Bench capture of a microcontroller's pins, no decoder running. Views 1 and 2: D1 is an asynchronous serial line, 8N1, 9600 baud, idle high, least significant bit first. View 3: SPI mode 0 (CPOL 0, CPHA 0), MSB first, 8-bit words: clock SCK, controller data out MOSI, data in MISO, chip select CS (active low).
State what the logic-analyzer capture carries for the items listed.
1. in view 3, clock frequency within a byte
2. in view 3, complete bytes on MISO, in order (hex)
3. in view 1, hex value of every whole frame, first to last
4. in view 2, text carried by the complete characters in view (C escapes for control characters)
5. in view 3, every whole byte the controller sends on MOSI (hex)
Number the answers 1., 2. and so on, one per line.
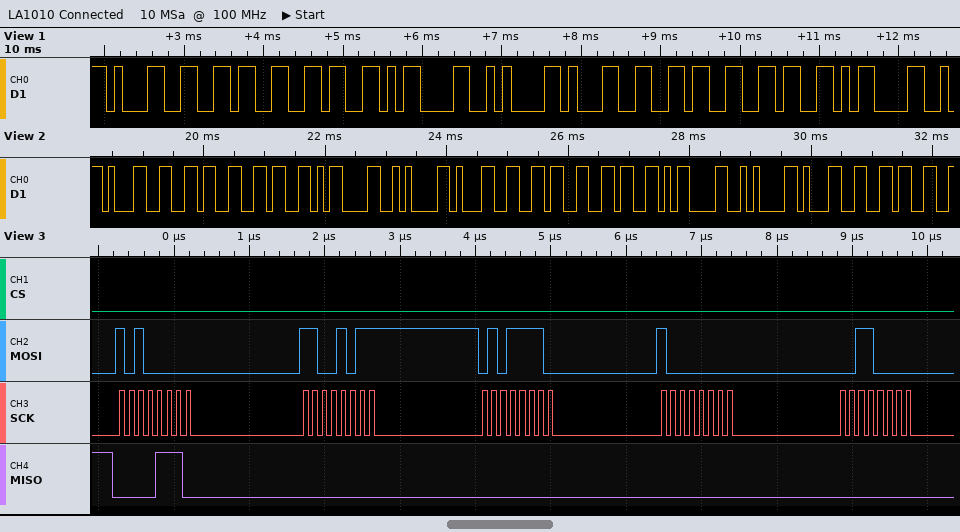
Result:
1. 8 MHz
2. 0E 00 00 00 00
3. 0x31 0x36 0x36 0x0D 0x0A 0x31 0x36 0x36 0x0D
4. "166\r\n166\r\n16"
5. A0 CB 5E 80 30
